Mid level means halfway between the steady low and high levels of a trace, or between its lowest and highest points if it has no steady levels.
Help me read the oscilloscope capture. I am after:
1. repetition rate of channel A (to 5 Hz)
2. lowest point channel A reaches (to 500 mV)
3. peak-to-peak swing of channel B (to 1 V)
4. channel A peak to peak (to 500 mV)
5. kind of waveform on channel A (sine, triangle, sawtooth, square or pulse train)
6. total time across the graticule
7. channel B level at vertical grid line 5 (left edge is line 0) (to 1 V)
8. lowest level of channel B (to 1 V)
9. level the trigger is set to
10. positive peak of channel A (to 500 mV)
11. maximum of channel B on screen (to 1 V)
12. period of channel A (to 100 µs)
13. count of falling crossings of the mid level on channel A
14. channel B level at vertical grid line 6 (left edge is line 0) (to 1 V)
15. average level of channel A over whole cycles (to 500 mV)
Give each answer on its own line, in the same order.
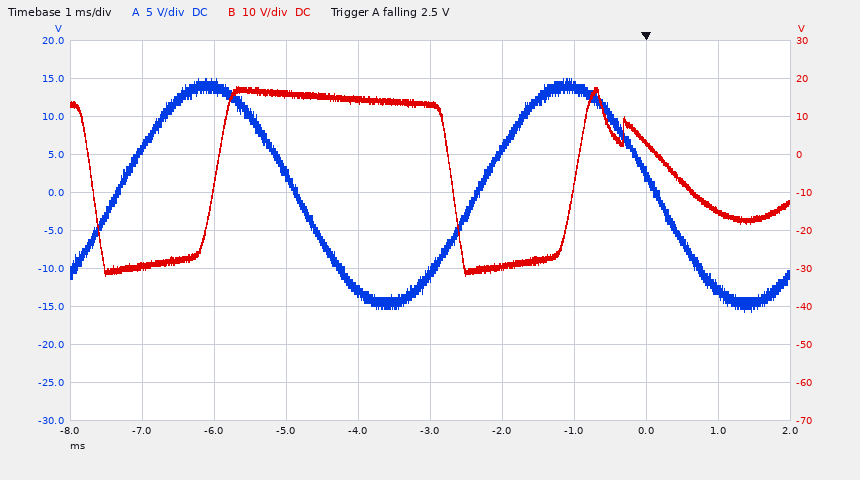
200 Hz
-16.0 V
50 V
31.0 V
sine
10 ms
13 V
-32 V
2.5 V
15.0 V
18 V
5.0 ms
2
-30 V
-500 mV
